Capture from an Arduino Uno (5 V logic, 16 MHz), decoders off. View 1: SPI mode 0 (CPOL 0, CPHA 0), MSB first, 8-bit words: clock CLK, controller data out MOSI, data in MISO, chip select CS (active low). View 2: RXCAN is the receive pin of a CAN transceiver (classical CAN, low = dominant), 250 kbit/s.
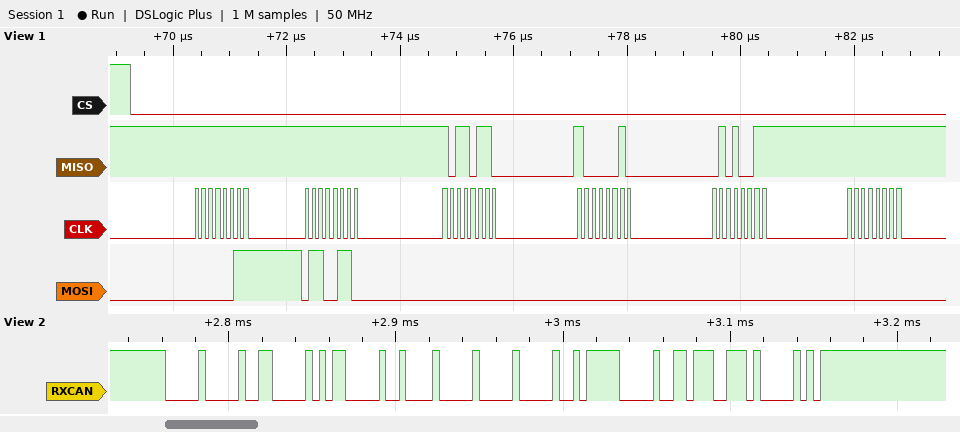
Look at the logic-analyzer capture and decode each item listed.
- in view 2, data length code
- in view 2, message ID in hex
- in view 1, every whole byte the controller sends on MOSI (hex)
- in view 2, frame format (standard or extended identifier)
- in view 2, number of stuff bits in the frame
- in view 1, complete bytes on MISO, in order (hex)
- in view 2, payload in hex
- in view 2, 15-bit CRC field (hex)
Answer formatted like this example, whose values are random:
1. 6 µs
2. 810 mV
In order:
1. 4
2. 0x00000B01
3. 03 66 00 00 00 00
4. extended
5. 10
6. FF FF B6 82 53 FF
7. 00 01 7C 0D
8. 0x6740
